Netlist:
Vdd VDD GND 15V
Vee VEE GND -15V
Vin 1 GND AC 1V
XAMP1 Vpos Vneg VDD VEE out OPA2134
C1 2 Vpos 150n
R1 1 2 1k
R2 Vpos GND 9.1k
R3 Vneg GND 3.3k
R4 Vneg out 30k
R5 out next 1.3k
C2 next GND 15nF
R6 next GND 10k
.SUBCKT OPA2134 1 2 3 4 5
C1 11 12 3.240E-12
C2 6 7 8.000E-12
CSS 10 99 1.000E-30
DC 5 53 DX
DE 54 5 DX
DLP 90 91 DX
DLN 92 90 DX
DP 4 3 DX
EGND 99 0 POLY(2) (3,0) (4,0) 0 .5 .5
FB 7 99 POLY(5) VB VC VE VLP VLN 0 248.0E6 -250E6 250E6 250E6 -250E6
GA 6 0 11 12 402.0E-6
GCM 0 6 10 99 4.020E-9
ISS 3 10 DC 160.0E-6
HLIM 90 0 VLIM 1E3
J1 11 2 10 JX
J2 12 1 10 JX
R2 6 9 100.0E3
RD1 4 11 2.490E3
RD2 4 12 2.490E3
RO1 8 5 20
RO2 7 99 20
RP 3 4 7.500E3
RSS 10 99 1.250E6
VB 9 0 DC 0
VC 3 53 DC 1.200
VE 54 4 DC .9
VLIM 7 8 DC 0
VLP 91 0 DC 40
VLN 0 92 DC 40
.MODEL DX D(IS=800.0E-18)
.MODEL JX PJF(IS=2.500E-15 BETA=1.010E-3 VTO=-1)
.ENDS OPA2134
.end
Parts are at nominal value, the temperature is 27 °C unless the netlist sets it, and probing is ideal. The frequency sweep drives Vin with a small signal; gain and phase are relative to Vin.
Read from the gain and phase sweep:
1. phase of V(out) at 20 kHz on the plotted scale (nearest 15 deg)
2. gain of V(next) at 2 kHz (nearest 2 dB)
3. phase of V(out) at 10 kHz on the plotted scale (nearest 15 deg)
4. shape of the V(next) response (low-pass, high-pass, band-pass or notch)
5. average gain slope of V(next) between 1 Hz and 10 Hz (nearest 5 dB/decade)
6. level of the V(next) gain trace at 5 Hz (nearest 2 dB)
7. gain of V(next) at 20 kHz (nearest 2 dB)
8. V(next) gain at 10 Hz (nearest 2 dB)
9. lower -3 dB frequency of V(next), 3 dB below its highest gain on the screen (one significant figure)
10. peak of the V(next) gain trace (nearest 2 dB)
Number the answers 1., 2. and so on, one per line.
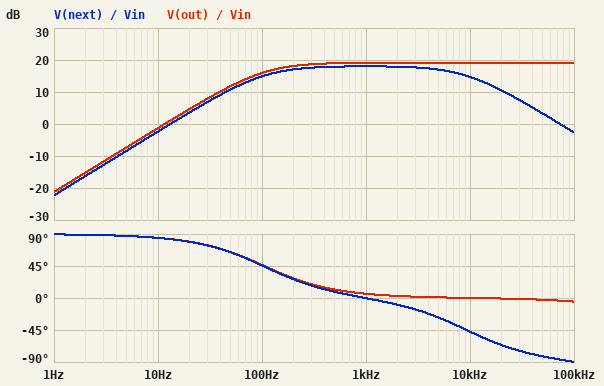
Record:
1. 0 deg
2. 18 dB
3. 0 deg
4. band-pass
5. 20 dB/decade
6. -8 dB
7. 10 dB
8. -2 dB
9. 100 Hz
10. 18 dB
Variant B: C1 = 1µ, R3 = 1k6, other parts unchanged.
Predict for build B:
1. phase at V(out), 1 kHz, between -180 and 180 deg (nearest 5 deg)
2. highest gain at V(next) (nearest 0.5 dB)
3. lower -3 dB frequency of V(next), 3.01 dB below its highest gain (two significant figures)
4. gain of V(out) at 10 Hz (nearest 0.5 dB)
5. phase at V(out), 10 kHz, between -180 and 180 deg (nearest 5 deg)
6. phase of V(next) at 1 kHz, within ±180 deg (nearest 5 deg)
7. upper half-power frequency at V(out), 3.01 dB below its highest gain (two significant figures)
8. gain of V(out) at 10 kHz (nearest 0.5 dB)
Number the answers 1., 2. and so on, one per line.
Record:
1. 0 deg
2. 24.0 dB
3. 16 Hz
4. 19.5 dB
5. 0 deg
6. -5 deg
7. 600 kHz
8. 25.0 dB
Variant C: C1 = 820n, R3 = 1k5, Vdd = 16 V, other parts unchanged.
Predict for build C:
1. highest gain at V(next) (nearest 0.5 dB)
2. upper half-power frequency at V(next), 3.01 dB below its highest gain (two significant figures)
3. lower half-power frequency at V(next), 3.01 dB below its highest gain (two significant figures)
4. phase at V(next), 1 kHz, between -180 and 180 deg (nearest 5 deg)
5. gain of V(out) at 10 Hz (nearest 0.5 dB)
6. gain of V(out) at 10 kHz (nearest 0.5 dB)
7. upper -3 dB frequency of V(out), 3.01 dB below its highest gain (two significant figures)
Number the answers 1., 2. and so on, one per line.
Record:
1. 24.5 dB
2. 9.3 kHz
3. 19 Hz
4. -5 deg
5. 19.0 dB
6. 25.5 dB
7. 560 kHz
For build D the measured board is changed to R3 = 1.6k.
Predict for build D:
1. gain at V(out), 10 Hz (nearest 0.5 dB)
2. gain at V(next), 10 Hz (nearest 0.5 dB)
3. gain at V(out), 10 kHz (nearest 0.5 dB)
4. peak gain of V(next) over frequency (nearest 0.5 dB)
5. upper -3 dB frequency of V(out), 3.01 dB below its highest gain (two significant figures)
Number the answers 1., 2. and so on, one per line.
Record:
1. 4.5 dB
2. 3.5 dB
3. 25.0 dB
4. 24.0 dB
5. 600 kHz
